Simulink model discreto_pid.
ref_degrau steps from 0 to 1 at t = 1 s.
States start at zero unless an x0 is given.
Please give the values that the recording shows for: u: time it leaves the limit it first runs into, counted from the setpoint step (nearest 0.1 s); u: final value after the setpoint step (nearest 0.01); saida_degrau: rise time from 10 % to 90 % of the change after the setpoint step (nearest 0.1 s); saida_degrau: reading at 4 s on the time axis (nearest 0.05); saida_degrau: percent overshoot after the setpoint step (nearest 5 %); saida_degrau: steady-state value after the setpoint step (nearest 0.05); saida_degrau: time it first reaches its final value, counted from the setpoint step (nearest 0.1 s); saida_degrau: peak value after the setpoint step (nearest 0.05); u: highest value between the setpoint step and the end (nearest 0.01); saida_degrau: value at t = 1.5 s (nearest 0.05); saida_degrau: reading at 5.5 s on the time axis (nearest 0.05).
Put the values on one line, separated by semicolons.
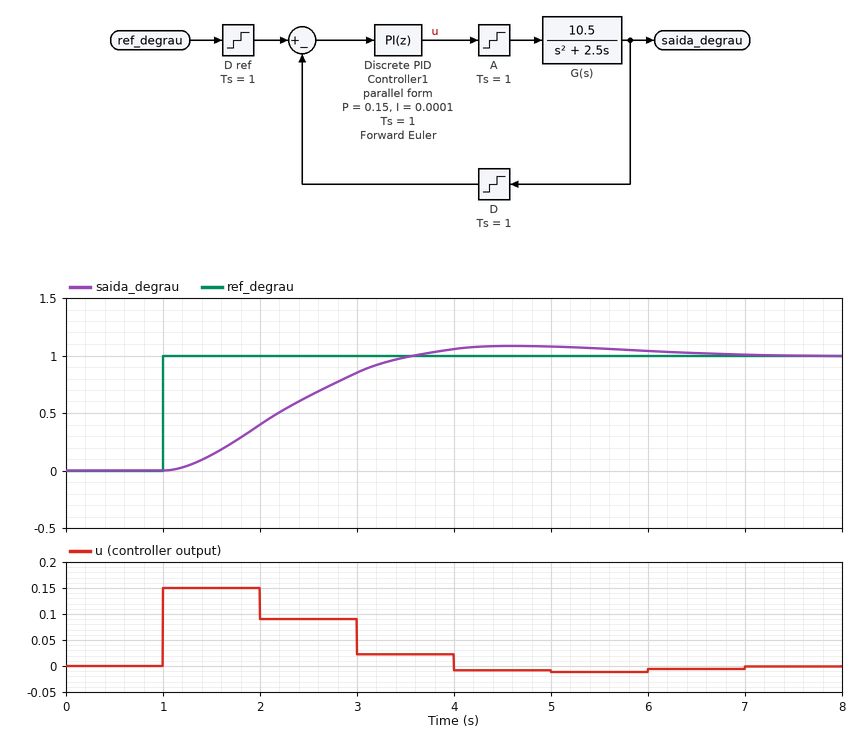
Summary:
1.0 s; 0.00; 1.7 s; 1.05; 10 %; 1.00; 2.6 s; 1.10; 0.15; 0.15; 1.05
